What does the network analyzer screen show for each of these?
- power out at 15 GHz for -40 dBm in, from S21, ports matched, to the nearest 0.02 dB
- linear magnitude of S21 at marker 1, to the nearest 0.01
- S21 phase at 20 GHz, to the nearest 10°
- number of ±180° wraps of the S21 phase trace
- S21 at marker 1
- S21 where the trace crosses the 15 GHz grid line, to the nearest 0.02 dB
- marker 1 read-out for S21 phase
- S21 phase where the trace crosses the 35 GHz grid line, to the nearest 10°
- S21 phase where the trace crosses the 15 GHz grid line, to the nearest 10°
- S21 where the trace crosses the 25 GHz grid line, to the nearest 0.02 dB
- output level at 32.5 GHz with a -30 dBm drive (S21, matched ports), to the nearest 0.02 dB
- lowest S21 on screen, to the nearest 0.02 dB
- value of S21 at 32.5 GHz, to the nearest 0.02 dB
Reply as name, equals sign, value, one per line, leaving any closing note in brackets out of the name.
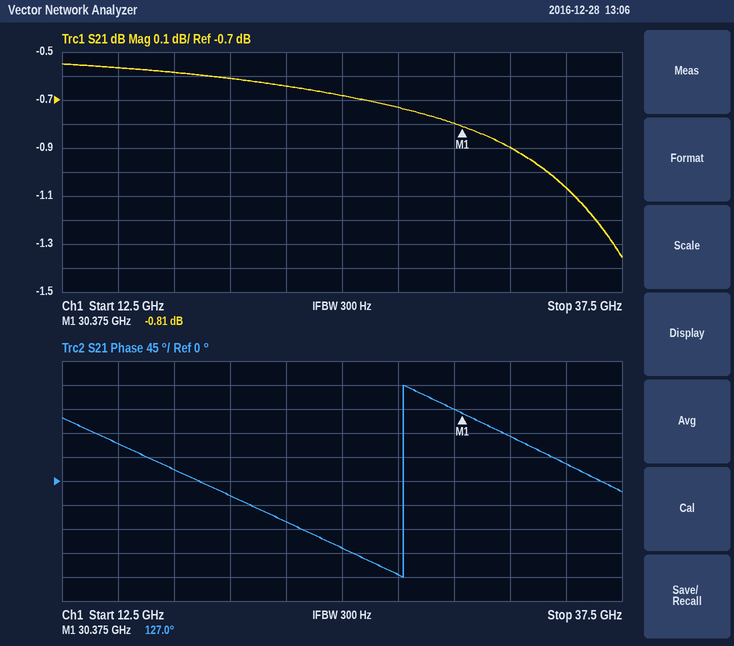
power out at 15 GHz for -40 dBm in, from S21, ports matched, to the nearest 0.02 dB = -40.56 dBm
linear magnitude of S21 at marker 1, to the nearest 0.01 = 0.91
S21 phase at 20 GHz, to the nearest 10° = -30°
number of ±180° wraps of the S21 phase trace = 1
S21 at marker 1 = -0.81 dB
S21 where the trace crosses the 15 GHz grid line, to the nearest 0.02 dB = -0.56 dB
marker 1 read-out for S21 phase = 127.0°
S21 phase where the trace crosses the 35 GHz grid line, to the nearest 10° = 30°
S21 phase where the trace crosses the 15 GHz grid line, to the nearest 10° = 70°
S21 where the trace crosses the 25 GHz grid line, to the nearest 0.02 dB = -0.68 dB
output level at 32.5 GHz with a -30 dBm drive (S21, matched ports), to the nearest 0.02 dB = -30.90 dBm
lowest S21 on screen, to the nearest 0.02 dB = -1.36 dB
value of S21 at 32.5 GHz, to the nearest 0.02 dB = -0.90 dB
